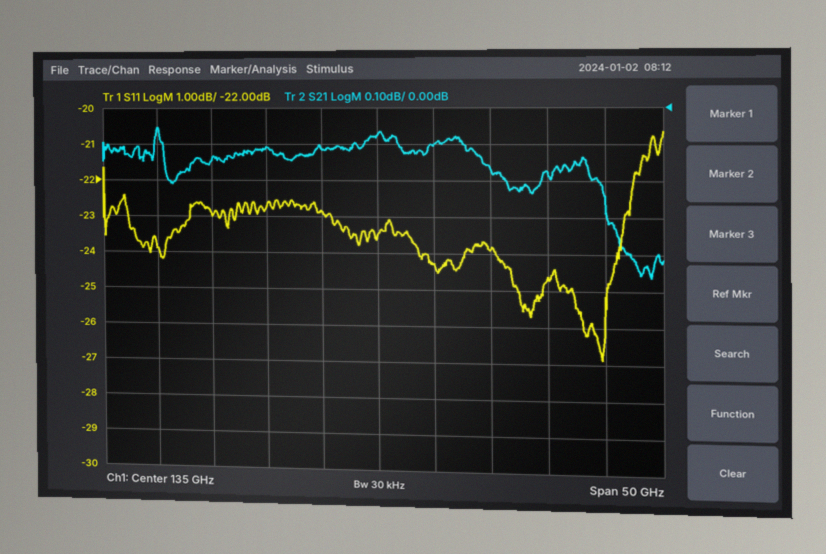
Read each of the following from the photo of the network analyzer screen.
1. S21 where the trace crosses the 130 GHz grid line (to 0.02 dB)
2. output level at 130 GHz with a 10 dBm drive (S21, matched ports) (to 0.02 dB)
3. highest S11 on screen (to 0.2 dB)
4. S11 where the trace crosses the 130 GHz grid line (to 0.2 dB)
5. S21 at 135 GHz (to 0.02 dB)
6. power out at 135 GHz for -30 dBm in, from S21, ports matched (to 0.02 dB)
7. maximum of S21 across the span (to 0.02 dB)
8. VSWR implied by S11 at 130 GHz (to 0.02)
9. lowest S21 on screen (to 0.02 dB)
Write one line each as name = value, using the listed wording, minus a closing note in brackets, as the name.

S21 where the trace crosses the 130 GHz grid line = -0.12 dB
output level at 130 GHz with a 10 dBm drive (S21, matched ports) = 9.88 dBm
highest S11 on screen = -20.6 dB
S11 where the trace crosses the 130 GHz grid line = -22.8 dB
S21 at 135 GHz = -0.08 dB
power out at 135 GHz for -30 dBm in, from S21, ports matched = -30.08 dBm
maximum of S21 across the span = -0.06 dB
VSWR implied by S11 at 130 GHz = 1.16
lowest S21 on screen = -0.46 dB
